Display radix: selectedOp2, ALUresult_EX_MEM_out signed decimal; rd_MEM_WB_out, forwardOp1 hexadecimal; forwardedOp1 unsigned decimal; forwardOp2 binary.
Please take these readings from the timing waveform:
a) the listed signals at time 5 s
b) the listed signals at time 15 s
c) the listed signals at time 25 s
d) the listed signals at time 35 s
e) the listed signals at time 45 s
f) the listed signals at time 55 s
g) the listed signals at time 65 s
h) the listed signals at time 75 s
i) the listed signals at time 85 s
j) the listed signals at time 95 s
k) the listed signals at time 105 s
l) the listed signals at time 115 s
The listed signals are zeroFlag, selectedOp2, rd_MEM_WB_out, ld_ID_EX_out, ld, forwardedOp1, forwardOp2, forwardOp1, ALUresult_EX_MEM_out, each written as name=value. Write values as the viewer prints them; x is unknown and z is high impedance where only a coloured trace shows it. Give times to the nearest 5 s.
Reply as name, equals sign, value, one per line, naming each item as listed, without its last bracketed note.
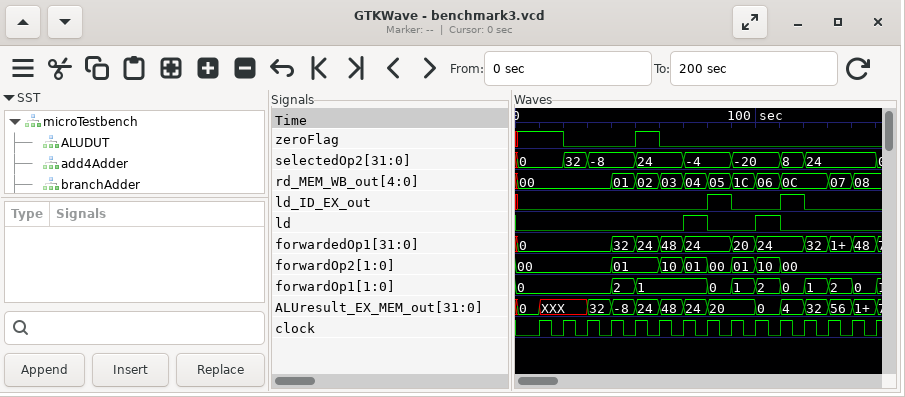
the listed signals at time 5 s = zeroFlag=1, selectedOp2=0, rd_MEM_WB_out=00, ld_ID_EX_out=0, ld=0, forwardedOp1=0, forwardOp2=00, forwardOp1=0, ALUresult_EX_MEM_out=0
the listed signals at time 15 s = zeroFlag=1, selectedOp2=0, rd_MEM_WB_out=00, ld_ID_EX_out=0, ld=0, forwardedOp1=0, forwardOp2=00, forwardOp1=0, ALUresult_EX_MEM_out=XXX
the listed signals at time 25 s = zeroFlag=0, selectedOp2=32, rd_MEM_WB_out=00, ld_ID_EX_out=0, ld=0, forwardedOp1=0, forwardOp2=00, forwardOp1=0, ALUresult_EX_MEM_out=XXX
the listed signals at time 35 s = zeroFlag=0, selectedOp2=-8, rd_MEM_WB_out=00, ld_ID_EX_out=0, ld=0, forwardedOp1=0, forwardOp2=00, forwardOp1=0, ALUresult_EX_MEM_out=32
the listed signals at time 45 s = zeroFlag=0, selectedOp2=-8, rd_MEM_WB_out=01, ld_ID_EX_out=0, ld=0, forwardedOp1=32, forwardOp2=01, forwardOp1=2, ALUresult_EX_MEM_out=-8
the listed signals at time 55 s = zeroFlag=1, selectedOp2=24, rd_MEM_WB_out=02, ld_ID_EX_out=0, ld=0, forwardedOp1=24, forwardOp2=01, forwardOp1=1, ALUresult_EX_MEM_out=24
the listed signals at time 65 s = zeroFlag=0, selectedOp2=24, rd_MEM_WB_out=03, ld_ID_EX_out=0, ld=0, forwardedOp1=48, forwardOp2=10, forwardOp1=1, ALUresult_EX_MEM_out=48
the listed signals at time 75 s = zeroFlag=0, selectedOp2=-4, rd_MEM_WB_out=04, ld_ID_EX_out=0, ld=1, forwardedOp1=24, forwardOp2=01, forwardOp1=1, ALUresult_EX_MEM_out=24
the listed signals at time 85 s = zeroFlag=0, selectedOp2=-4, rd_MEM_WB_out=05, ld_ID_EX_out=1, ld=0, forwardedOp1=24, forwardOp2=00, forwardOp1=0, ALUresult_EX_MEM_out=20
the listed signals at time 95 s = zeroFlag=0, selectedOp2=-20, rd_MEM_WB_out=1C, ld_ID_EX_out=0, ld=0, forwardedOp1=20, forwardOp2=01, forwardOp1=1, ALUresult_EX_MEM_out=20
the listed signals at time 105 s = zeroFlag=0, selectedOp2=-20, rd_MEM_WB_out=06, ld_ID_EX_out=0, ld=1, forwardedOp1=24, forwardOp2=10, forwardOp1=2, ALUresult_EX_MEM_out=0
the listed signals at time 115 s = zeroFlag=0, selectedOp2=8, rd_MEM_WB_out=0C, ld_ID_EX_out=1, ld=0, forwardedOp1=24, forwardOp2=00, forwardOp1=0, ALUresult_EX_MEM_out=4
